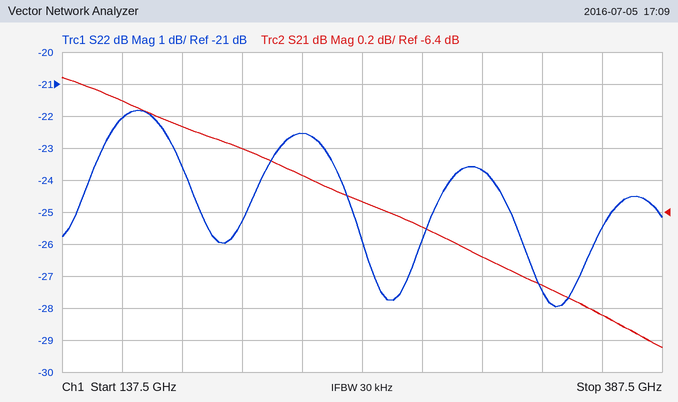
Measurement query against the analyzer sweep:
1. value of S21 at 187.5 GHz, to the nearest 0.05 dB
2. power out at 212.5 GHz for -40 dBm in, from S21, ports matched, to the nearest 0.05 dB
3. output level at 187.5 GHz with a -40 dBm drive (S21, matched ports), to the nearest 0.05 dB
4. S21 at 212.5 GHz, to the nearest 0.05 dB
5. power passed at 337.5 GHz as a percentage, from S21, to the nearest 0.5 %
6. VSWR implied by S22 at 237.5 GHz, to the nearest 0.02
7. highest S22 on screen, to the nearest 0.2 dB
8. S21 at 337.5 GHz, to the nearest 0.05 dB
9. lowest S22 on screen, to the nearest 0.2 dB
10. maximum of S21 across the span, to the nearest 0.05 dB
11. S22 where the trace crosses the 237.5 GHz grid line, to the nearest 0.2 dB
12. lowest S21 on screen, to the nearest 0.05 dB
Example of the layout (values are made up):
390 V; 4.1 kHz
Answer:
-5.85 dB; -46.00 dBm; -45.85 dBm; -6.00 dB; 20.5 %; 1.16; -21.8 dB; -6.85 dB; -28.0 dB; -5.55 dB; -22.6 dB; -7.25 dB
